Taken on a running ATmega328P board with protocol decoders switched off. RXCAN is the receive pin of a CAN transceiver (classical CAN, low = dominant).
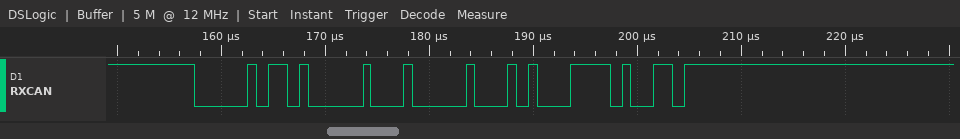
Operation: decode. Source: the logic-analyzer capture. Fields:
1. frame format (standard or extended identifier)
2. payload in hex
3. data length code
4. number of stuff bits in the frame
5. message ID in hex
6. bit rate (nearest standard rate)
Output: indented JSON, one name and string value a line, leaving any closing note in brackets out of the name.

{
  "frame format": "standard",
  "payload in hex": "00",
  "data length code": "1",
  "number of stuff bits in the frame": "3",
  "message ID in hex": "0x034",
  "bit rate": "1000 kbit/s"
}
